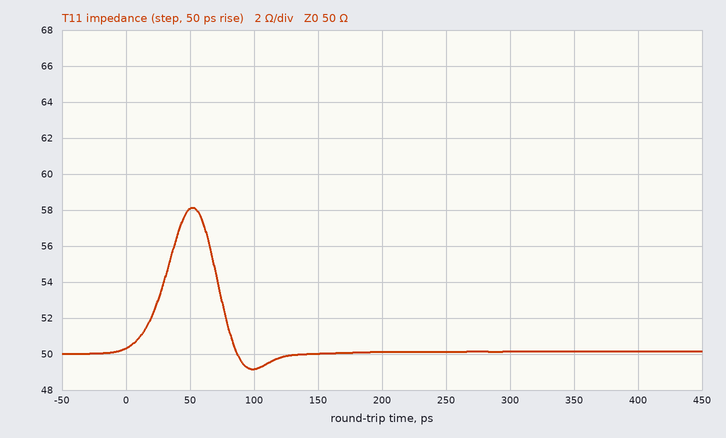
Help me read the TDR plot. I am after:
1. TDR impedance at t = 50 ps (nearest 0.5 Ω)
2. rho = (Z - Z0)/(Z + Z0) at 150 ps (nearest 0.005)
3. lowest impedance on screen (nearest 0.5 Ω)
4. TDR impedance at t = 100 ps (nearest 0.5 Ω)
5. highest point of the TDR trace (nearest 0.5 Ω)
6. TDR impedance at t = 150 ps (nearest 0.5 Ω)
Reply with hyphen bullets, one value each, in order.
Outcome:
- 58.0 Ω
- 0.000
- 49.0 Ω
- 49.0 Ω
- 58.0 Ω
- 50.0 Ω
